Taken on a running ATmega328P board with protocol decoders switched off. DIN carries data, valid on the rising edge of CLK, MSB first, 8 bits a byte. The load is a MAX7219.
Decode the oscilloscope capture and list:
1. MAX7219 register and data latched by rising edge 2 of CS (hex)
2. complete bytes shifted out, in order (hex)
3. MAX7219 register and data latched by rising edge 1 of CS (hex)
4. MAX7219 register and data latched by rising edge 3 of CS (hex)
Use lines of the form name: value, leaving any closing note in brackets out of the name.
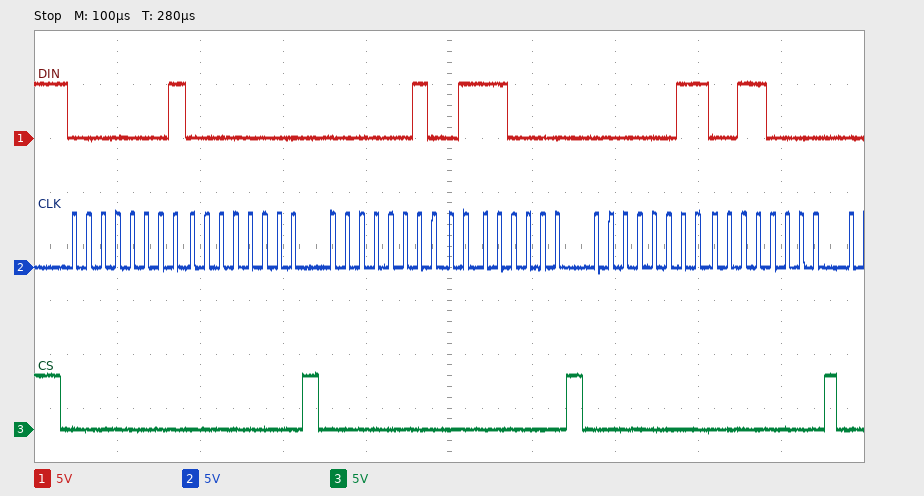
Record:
MAX7219 register and data latched by rising edge 2 of CS: register 0x2, data 0x70
complete bytes shifted out, in order: 01 00 02 70 03 30
MAX7219 register and data latched by rising edge 1 of CS: register 0x1, data 0x00
MAX7219 register and data latched by rising edge 3 of CS: register 0x3, data 0x30
